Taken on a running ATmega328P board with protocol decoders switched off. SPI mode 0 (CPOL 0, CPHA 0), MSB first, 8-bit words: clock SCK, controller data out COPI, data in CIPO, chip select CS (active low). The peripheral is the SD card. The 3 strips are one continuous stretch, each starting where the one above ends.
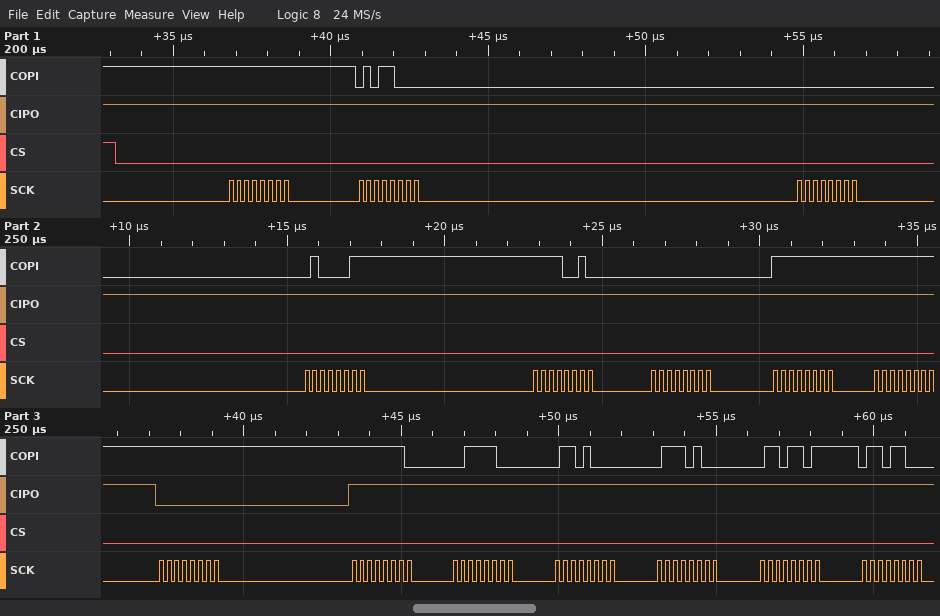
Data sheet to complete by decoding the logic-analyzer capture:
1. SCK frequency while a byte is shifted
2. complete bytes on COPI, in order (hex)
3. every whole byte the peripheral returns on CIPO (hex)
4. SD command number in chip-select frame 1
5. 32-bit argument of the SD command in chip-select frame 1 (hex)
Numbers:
4 MHz
FF 58 00 43 F2 00 FF FF FF FE 3C 68 74 6D 6C
FF FF FF FF FF FF FF FF 00 FF FF FF FF FF FF
CMD24
0x0043F200
